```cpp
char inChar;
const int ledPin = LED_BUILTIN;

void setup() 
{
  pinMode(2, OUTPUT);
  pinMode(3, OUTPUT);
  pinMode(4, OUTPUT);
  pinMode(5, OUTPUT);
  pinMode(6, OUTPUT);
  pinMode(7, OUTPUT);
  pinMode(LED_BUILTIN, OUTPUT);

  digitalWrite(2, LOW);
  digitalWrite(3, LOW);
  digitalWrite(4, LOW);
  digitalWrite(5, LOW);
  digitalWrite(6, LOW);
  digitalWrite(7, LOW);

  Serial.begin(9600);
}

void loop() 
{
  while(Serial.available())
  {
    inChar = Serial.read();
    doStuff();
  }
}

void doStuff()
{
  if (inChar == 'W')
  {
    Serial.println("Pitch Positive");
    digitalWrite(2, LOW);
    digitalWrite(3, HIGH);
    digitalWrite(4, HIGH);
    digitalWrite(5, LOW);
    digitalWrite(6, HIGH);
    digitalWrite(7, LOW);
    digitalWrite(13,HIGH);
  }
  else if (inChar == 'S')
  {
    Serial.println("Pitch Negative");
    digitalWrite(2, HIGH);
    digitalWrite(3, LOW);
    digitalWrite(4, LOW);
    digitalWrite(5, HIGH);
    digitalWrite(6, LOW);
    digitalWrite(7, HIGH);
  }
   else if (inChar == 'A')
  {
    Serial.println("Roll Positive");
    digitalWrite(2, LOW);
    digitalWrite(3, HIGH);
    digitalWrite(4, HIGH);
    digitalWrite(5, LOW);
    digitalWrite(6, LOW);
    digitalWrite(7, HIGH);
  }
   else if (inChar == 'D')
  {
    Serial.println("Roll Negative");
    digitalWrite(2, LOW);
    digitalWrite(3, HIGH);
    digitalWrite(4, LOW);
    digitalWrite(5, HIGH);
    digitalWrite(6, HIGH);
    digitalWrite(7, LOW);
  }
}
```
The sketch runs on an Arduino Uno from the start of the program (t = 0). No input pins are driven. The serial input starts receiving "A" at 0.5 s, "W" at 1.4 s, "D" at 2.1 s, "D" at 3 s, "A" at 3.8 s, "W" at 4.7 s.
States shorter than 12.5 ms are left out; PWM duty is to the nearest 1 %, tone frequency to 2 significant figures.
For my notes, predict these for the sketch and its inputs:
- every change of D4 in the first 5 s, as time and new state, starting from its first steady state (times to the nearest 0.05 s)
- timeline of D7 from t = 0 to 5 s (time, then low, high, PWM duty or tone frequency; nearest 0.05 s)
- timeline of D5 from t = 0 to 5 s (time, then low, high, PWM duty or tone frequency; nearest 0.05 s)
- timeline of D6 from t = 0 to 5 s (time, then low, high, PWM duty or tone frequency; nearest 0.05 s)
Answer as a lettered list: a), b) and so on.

a) 0 s low; 0.5 s high; 2.1 s low; 3.8 s high
b) 0 s low; 0.5 s high; 1.4 s low; 3.8 s high; 4.7 s low
c) 0 s low; 2.1 s high; 3.8 s low
d) 0 s low; 1.4 s high; 3.8 s low; 4.7 s high
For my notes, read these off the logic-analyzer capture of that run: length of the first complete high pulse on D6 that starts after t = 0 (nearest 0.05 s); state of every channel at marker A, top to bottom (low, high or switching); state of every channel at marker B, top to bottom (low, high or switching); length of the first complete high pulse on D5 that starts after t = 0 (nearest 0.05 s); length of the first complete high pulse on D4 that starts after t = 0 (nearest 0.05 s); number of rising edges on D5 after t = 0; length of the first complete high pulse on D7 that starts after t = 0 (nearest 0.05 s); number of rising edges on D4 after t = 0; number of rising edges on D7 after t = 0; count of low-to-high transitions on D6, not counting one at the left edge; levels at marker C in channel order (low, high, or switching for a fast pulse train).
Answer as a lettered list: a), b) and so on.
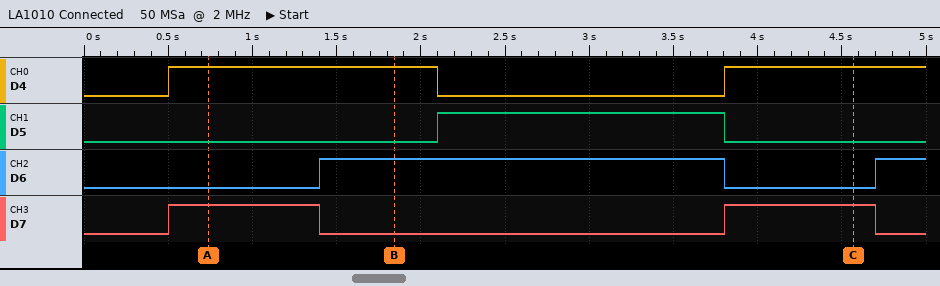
a) 2.40 s
b) D4 high, D5 low, D6 low, D7 high
c) D4 high, D5 low, D6 high, D7 low
d) 1.70 s
e) 1.60 s
f) 1
g) 0.90 s
h) 2
i) 2
j) 2
k) D4 high, D5 low, D6 low, D7 high
